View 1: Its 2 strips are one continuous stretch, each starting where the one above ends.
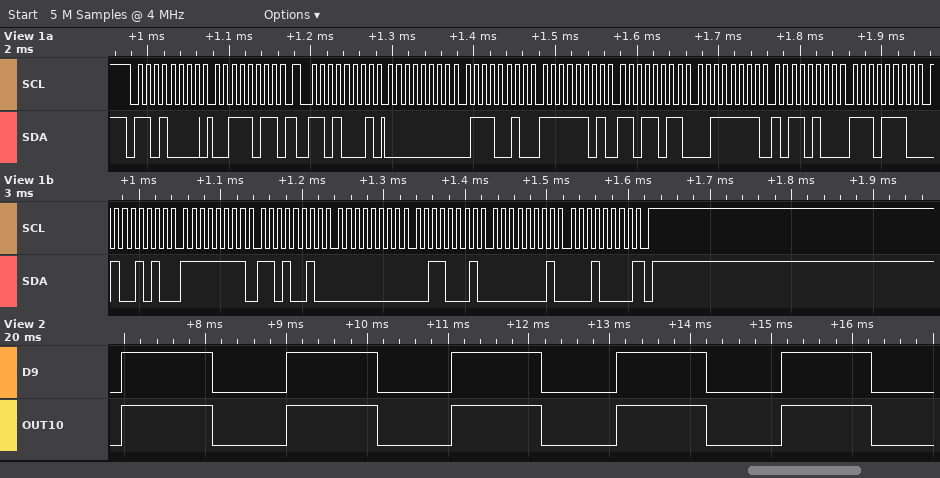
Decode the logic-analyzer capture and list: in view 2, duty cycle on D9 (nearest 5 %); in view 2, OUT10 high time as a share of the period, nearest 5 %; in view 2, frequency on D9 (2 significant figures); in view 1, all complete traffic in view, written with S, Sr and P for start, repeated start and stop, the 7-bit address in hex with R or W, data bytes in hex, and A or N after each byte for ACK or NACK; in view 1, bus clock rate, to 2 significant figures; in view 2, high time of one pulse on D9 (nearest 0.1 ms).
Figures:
55 %
55 %
490 Hz
S 68W A 3B A Sr 68R A 00 A 72 A FD A DB A 3F A B4 A EE A 4A A FF A D2 A 00 A 31 A 01 A 10 N P
100 kHz
1.1 ms
